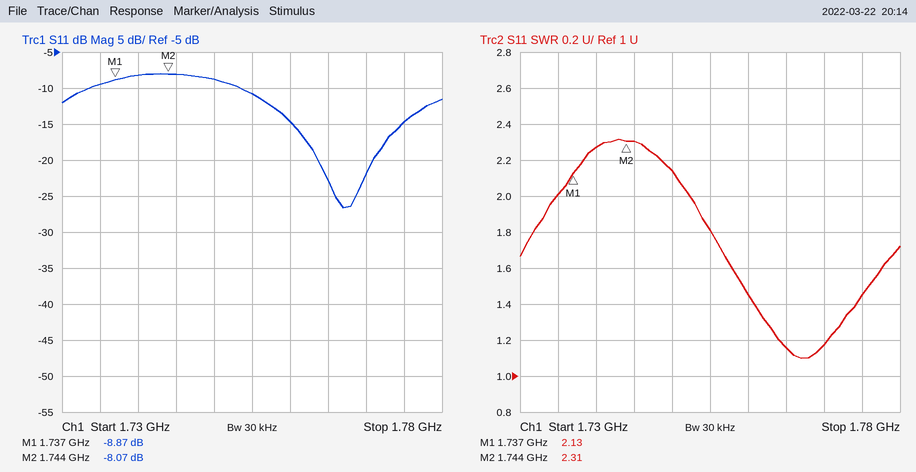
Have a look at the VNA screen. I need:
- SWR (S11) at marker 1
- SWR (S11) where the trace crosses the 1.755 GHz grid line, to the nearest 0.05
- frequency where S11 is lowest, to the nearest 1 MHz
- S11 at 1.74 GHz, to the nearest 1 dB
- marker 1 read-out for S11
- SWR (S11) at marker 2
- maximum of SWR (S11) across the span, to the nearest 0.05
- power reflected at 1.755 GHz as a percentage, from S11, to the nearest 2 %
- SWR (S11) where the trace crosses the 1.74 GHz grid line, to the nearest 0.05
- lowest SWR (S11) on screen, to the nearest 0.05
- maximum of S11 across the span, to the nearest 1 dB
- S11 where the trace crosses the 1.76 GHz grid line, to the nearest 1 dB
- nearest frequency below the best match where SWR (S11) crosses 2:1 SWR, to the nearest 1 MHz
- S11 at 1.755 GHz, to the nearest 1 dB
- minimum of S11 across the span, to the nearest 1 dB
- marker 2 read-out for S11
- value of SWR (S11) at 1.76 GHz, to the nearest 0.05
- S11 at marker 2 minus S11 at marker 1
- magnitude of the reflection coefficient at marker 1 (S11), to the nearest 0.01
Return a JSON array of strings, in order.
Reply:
["2.13", "1.80", "1.767 GHz", "-8 dB", "-8.87 dB", "2.31", "2.30", "8 %", "2.25", "1.10", "-8 dB", "-15 dB", "1.752 GHz", "-11 dB", "-27 dB", "-8.07 dB", "1.45", "0.80 dB", "0.36"]
